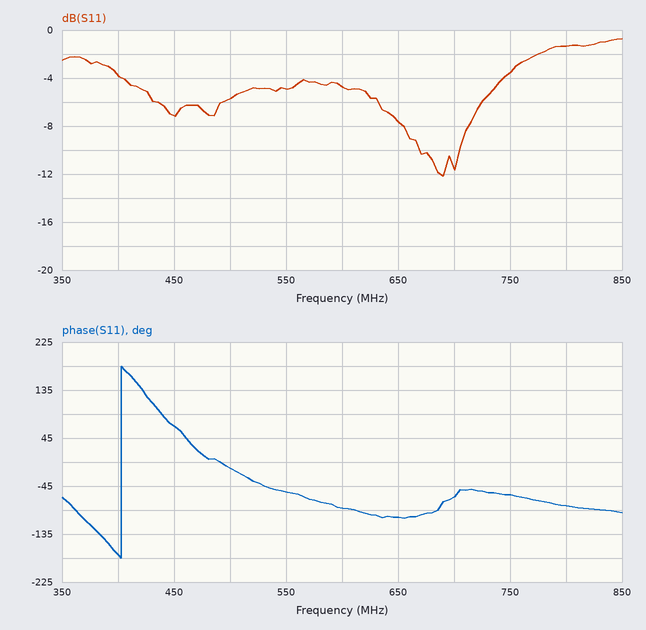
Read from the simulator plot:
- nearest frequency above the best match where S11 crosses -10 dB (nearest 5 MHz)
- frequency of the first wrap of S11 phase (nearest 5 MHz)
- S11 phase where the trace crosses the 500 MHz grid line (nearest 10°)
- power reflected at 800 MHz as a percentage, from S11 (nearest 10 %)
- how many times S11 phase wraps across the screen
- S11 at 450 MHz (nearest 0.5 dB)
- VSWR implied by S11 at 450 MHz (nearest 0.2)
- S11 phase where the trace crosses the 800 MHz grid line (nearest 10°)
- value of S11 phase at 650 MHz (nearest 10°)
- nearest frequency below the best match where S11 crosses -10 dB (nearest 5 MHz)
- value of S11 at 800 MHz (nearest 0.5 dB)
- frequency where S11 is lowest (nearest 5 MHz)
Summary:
705 MHz
405 MHz
-10°
70 %
1
-7.0 dB
2.6
-80°
-100°
670 MHz
-1.5 dB
690 MHz
